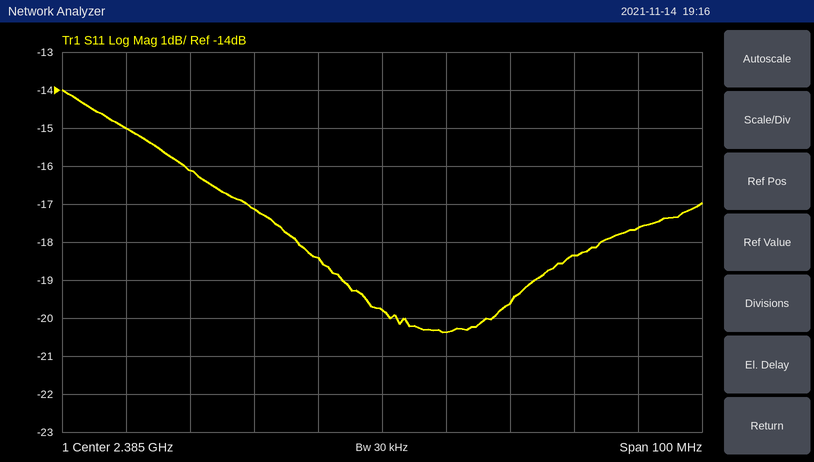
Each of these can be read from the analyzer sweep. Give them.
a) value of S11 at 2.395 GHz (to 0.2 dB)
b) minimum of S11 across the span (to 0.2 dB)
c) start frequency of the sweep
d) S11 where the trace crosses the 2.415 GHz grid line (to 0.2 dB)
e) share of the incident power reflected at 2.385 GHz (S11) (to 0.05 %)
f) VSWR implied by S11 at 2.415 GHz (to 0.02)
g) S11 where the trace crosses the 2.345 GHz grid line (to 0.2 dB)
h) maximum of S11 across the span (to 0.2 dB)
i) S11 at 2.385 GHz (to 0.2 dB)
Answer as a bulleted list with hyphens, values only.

- -20.4 dB
- -20.4 dB
- 2.335 GHz
- -18.4 dB
- 1.05 %
- 1.28
- -15.0 dB
- -14.0 dB
- -19.8 dB
